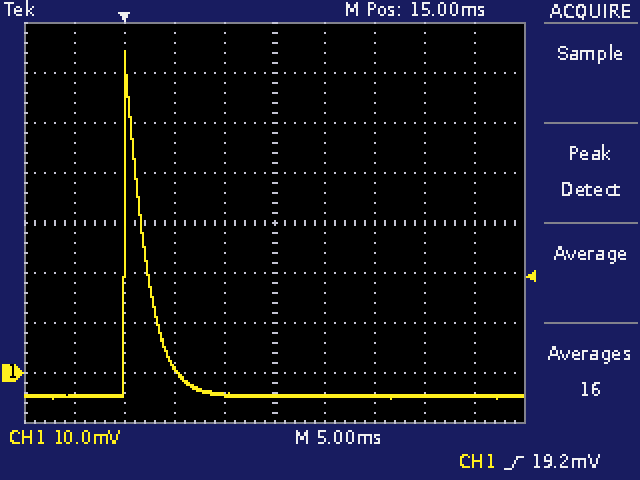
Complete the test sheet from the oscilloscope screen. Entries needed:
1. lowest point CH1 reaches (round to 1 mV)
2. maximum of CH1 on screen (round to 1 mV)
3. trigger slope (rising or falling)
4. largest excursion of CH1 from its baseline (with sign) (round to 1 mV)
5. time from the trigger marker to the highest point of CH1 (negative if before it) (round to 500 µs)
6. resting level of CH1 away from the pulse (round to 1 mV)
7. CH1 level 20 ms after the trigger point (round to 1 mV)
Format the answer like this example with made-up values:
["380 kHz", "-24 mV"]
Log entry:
["-5 mV", "64 mV", "rising", "+69 mV", "0.0 ms", "-5 mV", "-5 mV"]
